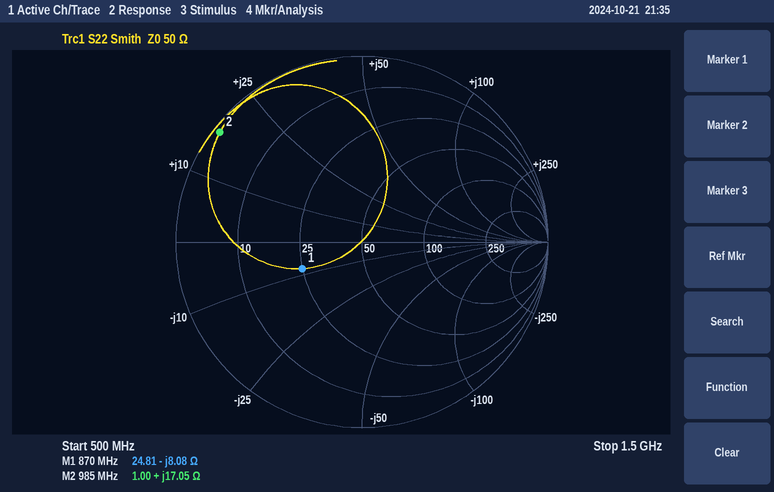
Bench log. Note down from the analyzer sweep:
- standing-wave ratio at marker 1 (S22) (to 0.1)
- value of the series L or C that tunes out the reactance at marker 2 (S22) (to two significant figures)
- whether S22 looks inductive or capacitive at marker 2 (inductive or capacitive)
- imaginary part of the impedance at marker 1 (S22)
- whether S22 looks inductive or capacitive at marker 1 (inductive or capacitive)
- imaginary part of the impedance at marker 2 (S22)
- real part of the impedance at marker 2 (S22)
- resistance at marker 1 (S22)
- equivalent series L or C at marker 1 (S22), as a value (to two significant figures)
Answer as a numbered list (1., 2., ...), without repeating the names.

1. 2.1
2. 9.5 pF
3. inductive
4. -8.08 Ω
5. capacitive
6. +17.05 Ω
7. 1.00 Ω
8. 24.81 Ω
9. 23 pF
